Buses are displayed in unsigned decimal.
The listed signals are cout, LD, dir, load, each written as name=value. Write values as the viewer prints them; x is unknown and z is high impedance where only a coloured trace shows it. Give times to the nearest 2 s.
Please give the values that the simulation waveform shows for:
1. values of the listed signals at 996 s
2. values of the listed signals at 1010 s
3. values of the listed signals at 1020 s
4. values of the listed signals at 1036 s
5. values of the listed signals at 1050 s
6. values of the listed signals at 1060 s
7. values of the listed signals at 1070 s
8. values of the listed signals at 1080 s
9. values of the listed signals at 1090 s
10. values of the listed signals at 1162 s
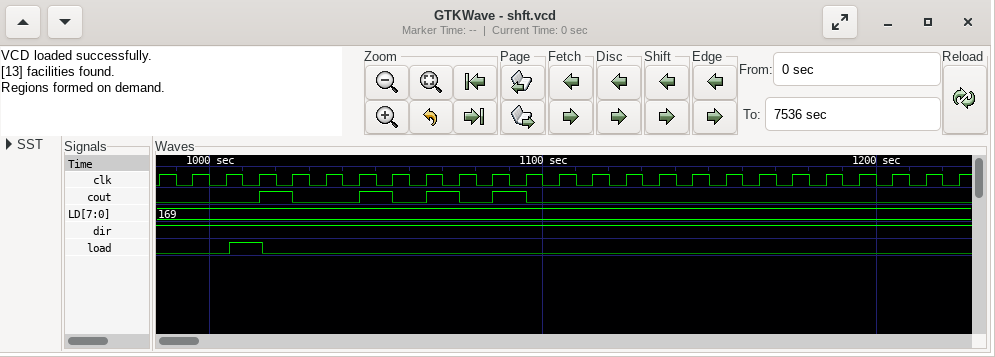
cout=0, LD=169, dir=1, load=0
cout=0, LD=169, dir=1, load=1
cout=1, LD=169, dir=1, load=0
cout=0, LD=169, dir=1, load=0
cout=1, LD=169, dir=1, load=0
cout=0, LD=169, dir=1, load=0
cout=1, LD=169, dir=1, load=0
cout=0, LD=169, dir=1, load=0
cout=1, LD=169, dir=1, load=0
cout=0, LD=169, dir=1, load=0
